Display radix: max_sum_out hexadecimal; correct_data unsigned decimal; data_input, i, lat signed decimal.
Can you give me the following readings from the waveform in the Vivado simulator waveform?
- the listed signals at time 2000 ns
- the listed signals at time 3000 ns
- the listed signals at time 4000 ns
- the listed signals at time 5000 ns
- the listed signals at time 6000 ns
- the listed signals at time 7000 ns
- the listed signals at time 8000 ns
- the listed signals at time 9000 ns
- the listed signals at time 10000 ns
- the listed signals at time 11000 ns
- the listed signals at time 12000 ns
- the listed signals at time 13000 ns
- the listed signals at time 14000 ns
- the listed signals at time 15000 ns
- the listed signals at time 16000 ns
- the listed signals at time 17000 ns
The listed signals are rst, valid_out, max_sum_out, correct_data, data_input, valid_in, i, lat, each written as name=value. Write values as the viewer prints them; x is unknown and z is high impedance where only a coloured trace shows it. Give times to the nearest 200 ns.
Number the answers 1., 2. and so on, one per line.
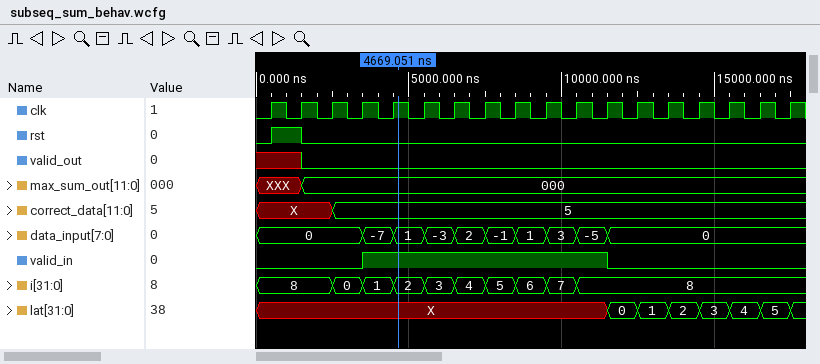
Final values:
1. rst=0, valid_out=0, max_sum_out=000, correct_data=X, data_input=0, valid_in=0, i=8, lat=X
2. rst=0, valid_out=0, max_sum_out=000, correct_data=5, data_input=0, valid_in=0, i=0, lat=X
3. rst=0, valid_out=0, max_sum_out=000, correct_data=5, data_input=-7, valid_in=1, i=1, lat=X
4. rst=0, valid_out=0, max_sum_out=000, correct_data=5, data_input=1, valid_in=1, i=2, lat=X
5. rst=0, valid_out=0, max_sum_out=000, correct_data=5, data_input=-3, valid_in=1, i=3, lat=X
6. rst=0, valid_out=0, max_sum_out=000, correct_data=5, data_input=2, valid_in=1, i=4, lat=X
7. rst=0, valid_out=0, max_sum_out=000, correct_data=5, data_input=-1, valid_in=1, i=5, lat=X
8. rst=0, valid_out=0, max_sum_out=000, correct_data=5, data_input=1, valid_in=1, i=6, lat=X
9. rst=0, valid_out=0, max_sum_out=000, correct_data=5, data_input=3, valid_in=1, i=7, lat=X
10. rst=0, valid_out=0, max_sum_out=000, correct_data=5, data_input=-5, valid_in=1, i=8, lat=X
11. rst=0, valid_out=0, max_sum_out=000, correct_data=5, data_input=0, valid_in=0, i=8, lat=0
12. rst=0, valid_out=0, max_sum_out=000, correct_data=5, data_input=0, valid_in=0, i=8, lat=1
13. rst=0, valid_out=0, max_sum_out=000, correct_data=5, data_input=0, valid_in=0, i=8, lat=2
14. rst=0, valid_out=0, max_sum_out=000, correct_data=5, data_input=0, valid_in=0, i=8, lat=3
15. rst=0, valid_out=0, max_sum_out=000, correct_data=5, data_input=0, valid_in=0, i=8, lat=4
16. rst=0, valid_out=0, max_sum_out=000, correct_data=5, data_input=0, valid_in=0, i=8, lat=5
